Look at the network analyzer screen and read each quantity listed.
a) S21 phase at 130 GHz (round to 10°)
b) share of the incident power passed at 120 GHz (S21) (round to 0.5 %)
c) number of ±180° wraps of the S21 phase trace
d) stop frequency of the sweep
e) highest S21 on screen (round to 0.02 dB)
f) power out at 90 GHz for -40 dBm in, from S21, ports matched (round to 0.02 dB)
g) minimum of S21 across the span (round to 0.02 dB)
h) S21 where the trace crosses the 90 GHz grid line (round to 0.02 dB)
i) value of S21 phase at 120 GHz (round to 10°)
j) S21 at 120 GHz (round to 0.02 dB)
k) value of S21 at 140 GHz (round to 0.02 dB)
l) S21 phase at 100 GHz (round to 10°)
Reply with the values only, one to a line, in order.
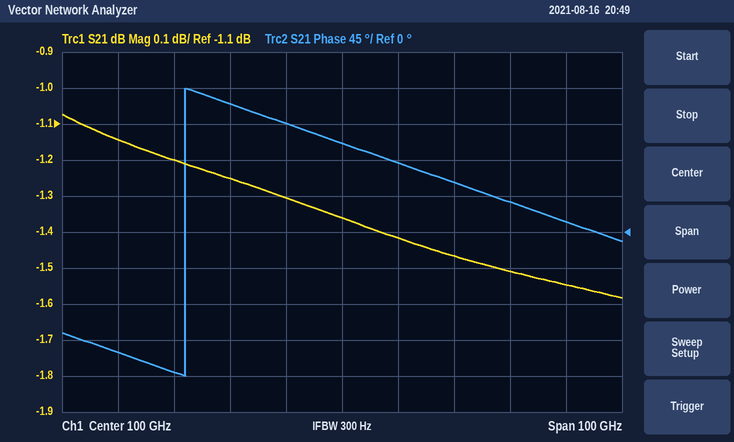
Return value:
40°
71.5 %
1
150 GHz
-1.08 dB
-41.30 dBm
-1.58 dB
-1.30 dB
60°
-1.46 dB
-1.54 dB
110°
